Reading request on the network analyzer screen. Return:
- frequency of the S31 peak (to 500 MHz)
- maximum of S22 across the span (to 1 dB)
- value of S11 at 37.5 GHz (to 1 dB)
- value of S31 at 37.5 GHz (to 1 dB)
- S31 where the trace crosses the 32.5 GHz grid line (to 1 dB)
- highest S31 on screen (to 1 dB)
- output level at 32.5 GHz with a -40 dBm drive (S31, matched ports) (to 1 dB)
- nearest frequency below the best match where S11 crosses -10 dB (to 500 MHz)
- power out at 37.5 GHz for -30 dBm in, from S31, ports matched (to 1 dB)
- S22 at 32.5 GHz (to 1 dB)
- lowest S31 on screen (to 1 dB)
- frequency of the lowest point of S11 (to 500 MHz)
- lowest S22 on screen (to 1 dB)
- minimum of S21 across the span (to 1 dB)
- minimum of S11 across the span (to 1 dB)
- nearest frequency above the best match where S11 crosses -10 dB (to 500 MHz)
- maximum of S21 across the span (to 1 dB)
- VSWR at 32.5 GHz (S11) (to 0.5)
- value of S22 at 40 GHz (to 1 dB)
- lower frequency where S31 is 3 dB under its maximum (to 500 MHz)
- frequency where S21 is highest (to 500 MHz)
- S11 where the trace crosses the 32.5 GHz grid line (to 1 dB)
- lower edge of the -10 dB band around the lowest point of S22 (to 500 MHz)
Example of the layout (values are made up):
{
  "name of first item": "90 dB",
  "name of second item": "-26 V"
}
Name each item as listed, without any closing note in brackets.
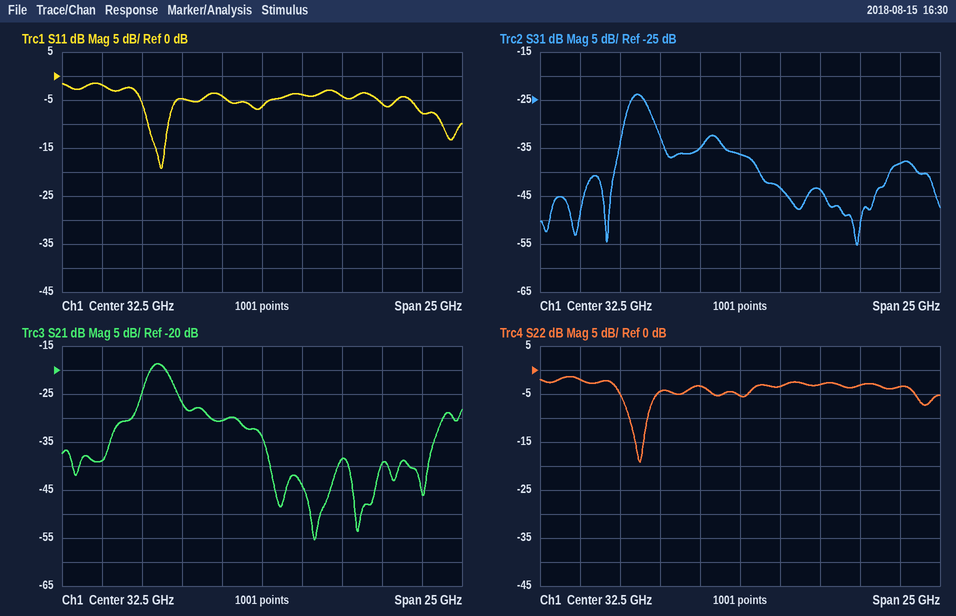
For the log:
{
  "frequency of the S31 peak": "26.0 GHz",
  "maximum of S22 across the span": "-1 dB",
  "value of S11 at 37.5 GHz": "-4 dB",
  "value of S31 at 37.5 GHz": "-44 dB",
  "S31 where the trace crosses the 32.5 GHz grid line": "-36 dB",
  "highest S31 on screen": "-24 dB",
  "output level at 32.5 GHz with a -40 dBm drive (S31, matched ports)": "-76 dBm",
  "nearest frequency below the best match where S11 crosses -10 dB": "25.5 GHz",
  "power out at 37.5 GHz for -30 dBm in, from S31, ports matched": "-74 dBm",
  "S22 at 32.5 GHz": "-5 dB",
  "lowest S31 on screen": "-55 dB",
  "frequency of the lowest point of S11": "26.0 GHz",
  "lowest S22 on screen": "-19 dB",
  "minimum of S21 across the span": "-55 dB",
  "minimum of S11 across the span": "-19 dB",
  "nearest frequency above the best match where S11 crosses -10 dB": "26.5 GHz",
  "maximum of S21 across the span": "-19 dB",
  "VSWR at 32.5 GHz (S11)": "3.0",
  "value of S22 at 40 GHz": "-3 dB",
  "lower frequency where S31 is 3 dB under its maximum": "25.5 GHz",
  "frequency where S21 is highest": "26.0 GHz",
  "S11 where the trace crosses the 32.5 GHz grid line": "-6 dB",
  "lower edge of the -10 dB band around the lowest point of S22": "25.5 GHz"
}
